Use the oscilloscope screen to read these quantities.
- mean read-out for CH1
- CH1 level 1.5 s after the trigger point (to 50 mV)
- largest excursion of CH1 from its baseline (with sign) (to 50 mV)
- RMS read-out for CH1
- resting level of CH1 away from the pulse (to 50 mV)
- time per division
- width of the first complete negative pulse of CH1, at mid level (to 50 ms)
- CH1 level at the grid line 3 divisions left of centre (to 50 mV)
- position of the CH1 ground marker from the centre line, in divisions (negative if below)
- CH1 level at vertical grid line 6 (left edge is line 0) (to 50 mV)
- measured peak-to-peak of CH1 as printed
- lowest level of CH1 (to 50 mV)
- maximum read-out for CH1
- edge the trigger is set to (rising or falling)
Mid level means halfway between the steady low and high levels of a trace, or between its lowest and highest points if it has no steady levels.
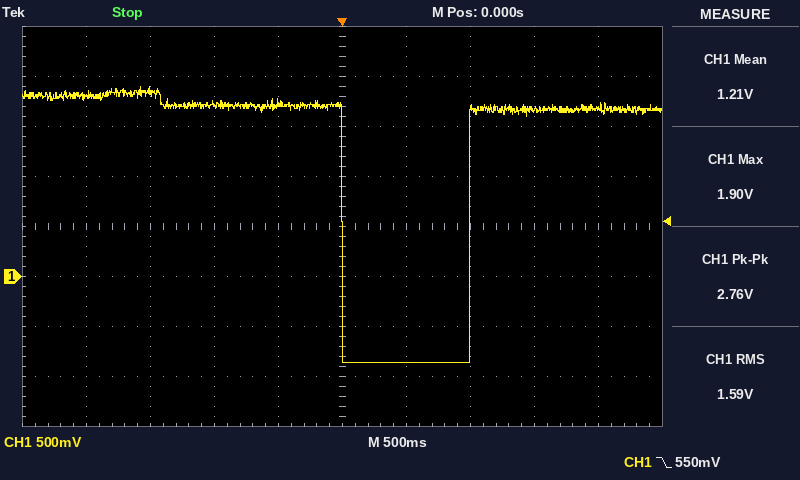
1.21 V
1.65 V
-2.55 V
1.59 V
1.70 V
500 ms
1.00 s
1.85 V
-1.0 div
-850 mV
2.76 V
-850 mV
1.90 V
falling
